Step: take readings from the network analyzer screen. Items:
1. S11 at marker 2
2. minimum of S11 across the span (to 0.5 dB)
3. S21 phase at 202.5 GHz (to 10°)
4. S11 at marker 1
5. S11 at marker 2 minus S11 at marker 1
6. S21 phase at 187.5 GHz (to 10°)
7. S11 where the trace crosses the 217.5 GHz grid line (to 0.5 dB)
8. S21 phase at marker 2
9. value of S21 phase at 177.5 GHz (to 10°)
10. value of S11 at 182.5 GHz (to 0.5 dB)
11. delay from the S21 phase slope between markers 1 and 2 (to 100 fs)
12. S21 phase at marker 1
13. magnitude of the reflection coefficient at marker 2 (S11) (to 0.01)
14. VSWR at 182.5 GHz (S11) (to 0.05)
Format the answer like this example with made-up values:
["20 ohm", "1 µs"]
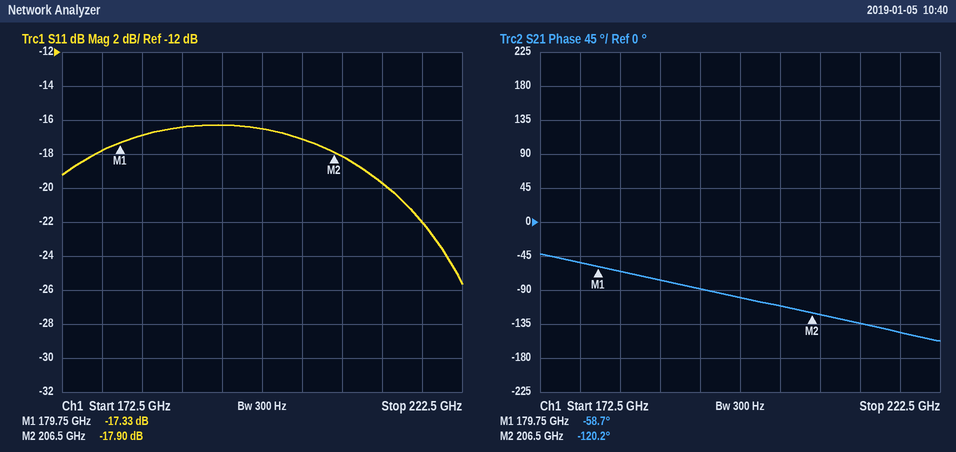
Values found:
["-17.90 dB", "-25.5 dB", "-110°", "-17.33 dB", "-0.57 dB", "-80°", "-22.0 dB", "-120.2°", "-50°", "-17.0 dB", "6.4 ps", "-58.7°", "0.13", "1.35"]
